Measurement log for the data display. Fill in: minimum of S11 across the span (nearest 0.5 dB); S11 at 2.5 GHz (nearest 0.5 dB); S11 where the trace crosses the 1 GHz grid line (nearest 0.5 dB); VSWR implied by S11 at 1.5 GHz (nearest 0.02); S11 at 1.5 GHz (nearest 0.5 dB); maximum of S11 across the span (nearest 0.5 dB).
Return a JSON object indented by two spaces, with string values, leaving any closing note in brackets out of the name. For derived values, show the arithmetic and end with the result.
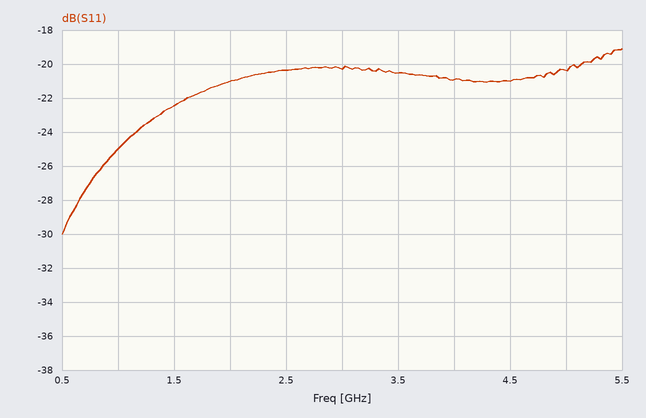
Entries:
{
  "minimum of S11 across the span": "-30.0 dB",
  "S11 at 2.5 GHz": "-20.5 dB",
  "S11 where the trace crosses the 1 GHz grid line": "-25.0 dB",
  "VSWR implied by S11 at 1.5 GHz": "|Γ| = 10^(-22.5/20) = 0.0750; VSWR = (1 + 0.0750)/(1 − 0.0750) ≈ 1.16",
  "S11 at 1.5 GHz": "-22.5 dB",
  "maximum of S11 across the span": "-19.0 dB"
}
